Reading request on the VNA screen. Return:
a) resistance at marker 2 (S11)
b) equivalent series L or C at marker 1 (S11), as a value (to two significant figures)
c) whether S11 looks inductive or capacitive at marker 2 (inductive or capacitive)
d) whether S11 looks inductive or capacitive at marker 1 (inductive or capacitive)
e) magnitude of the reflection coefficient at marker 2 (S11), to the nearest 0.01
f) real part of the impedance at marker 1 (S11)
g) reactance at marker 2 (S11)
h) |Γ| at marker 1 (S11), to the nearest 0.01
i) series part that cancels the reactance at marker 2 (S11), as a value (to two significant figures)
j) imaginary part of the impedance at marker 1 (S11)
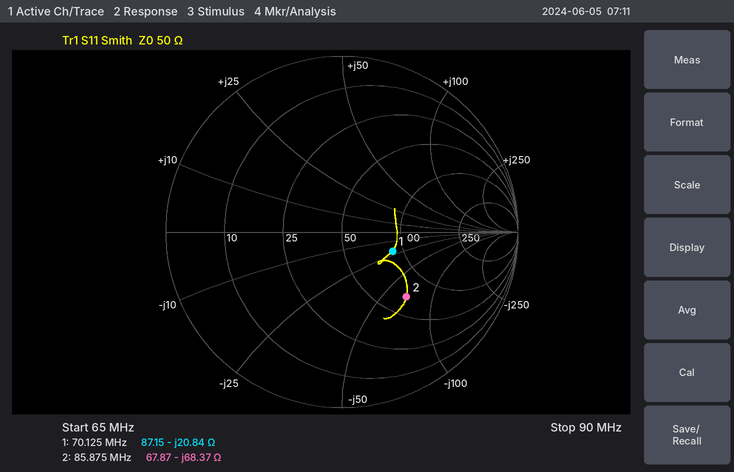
67.87 Ω
110 pF
capacitive
capacitive
0.52
87.15 Ω
-68.37 Ω
0.31
130 nH
-20.84 Ω
